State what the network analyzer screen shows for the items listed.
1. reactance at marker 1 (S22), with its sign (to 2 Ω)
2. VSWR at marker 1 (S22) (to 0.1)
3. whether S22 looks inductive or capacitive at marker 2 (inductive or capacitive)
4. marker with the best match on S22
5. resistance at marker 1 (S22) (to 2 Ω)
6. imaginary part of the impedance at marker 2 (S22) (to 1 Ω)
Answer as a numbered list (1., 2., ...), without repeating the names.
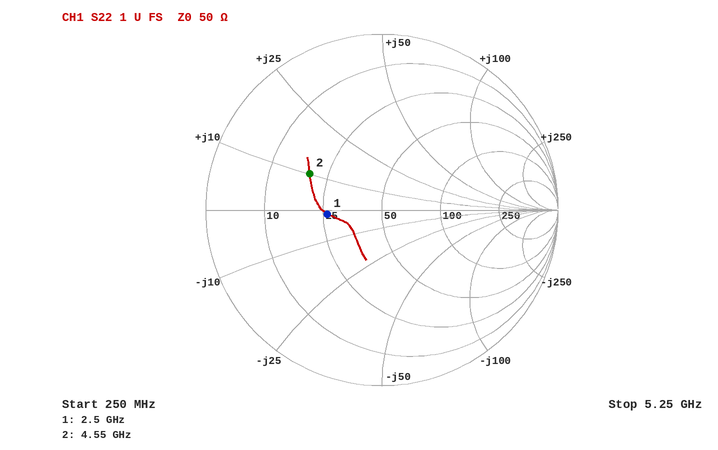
1. -2 Ω
2. 1.9
3. inductive
4. marker 1
5. 26 Ω
6. +10 Ω
